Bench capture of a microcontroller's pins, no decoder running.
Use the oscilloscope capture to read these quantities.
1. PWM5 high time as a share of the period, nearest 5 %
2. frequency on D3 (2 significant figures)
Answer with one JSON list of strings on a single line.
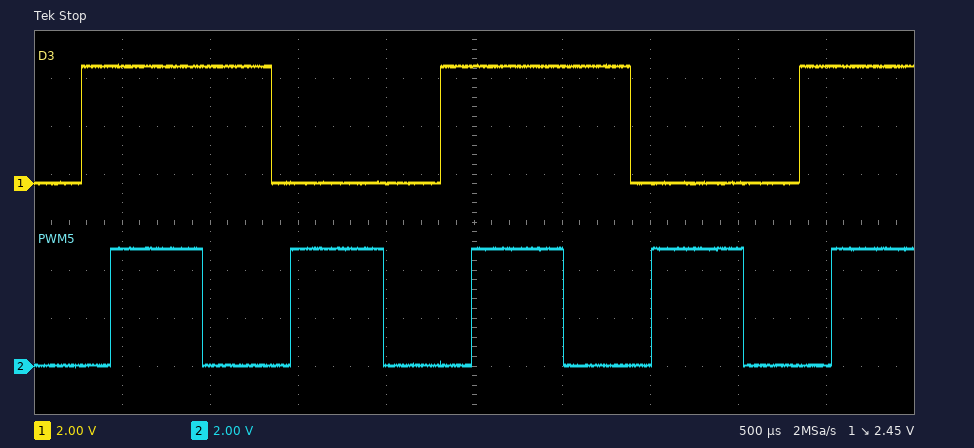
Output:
["50 %", "490 Hz"]
